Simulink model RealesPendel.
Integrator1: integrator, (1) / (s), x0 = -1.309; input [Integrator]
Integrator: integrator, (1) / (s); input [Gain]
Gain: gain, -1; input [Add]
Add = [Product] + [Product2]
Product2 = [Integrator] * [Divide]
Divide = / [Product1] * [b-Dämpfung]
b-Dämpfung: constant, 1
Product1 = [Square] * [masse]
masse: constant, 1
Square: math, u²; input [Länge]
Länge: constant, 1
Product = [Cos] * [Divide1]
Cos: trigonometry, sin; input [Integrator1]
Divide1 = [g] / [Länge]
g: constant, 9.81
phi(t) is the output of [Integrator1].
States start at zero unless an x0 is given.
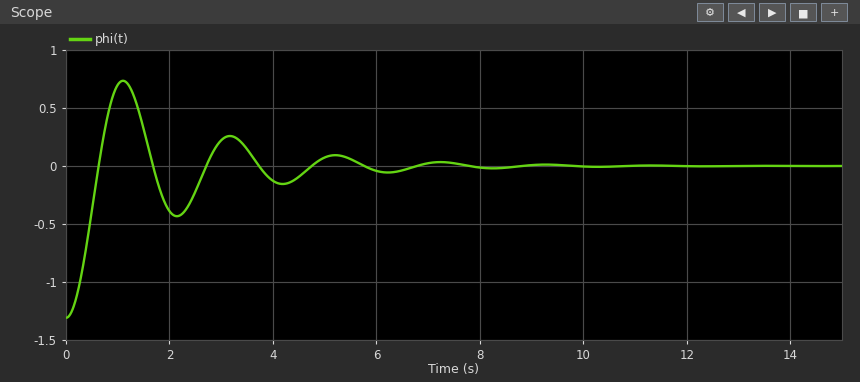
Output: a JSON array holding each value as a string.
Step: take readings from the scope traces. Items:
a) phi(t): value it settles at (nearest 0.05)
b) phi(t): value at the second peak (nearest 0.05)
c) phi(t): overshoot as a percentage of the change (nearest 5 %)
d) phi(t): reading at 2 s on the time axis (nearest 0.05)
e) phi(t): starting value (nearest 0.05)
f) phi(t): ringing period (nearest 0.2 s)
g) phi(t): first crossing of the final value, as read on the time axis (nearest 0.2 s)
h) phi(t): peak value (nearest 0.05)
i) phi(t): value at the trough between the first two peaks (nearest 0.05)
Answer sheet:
["0.00", "0.25", "55 %", "-0.40", "-1.30", "2.0 s", "0.6 s", "0.75", "-0.45"]
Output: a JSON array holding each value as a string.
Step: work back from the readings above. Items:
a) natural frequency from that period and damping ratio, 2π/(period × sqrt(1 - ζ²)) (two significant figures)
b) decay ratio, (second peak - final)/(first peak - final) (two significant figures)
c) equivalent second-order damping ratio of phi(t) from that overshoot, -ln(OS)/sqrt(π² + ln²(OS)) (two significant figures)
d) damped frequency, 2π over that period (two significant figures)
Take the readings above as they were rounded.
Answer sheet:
["3.2 rad/s", "0.33", "0.19", "3.1 rad/s"]
